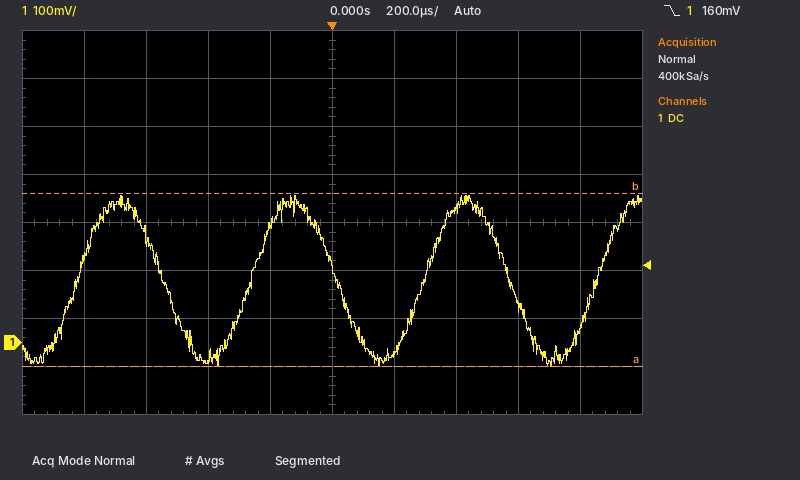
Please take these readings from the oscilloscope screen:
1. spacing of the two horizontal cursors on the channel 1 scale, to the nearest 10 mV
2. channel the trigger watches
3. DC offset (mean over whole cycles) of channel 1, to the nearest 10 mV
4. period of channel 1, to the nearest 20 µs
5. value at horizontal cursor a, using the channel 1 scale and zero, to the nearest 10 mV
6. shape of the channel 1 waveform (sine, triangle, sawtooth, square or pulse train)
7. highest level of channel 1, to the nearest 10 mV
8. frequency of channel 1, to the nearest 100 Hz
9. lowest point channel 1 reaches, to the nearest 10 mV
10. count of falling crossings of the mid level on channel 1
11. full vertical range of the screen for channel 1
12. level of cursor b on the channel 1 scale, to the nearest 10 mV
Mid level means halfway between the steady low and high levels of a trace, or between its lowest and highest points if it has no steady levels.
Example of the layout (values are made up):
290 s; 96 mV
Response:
360 mV; channel 1; 130 mV; 560 µs; -50 mV; sine; 310 mV; 1.8 kHz; -50 mV; 3; 800 mV; 310 mV
